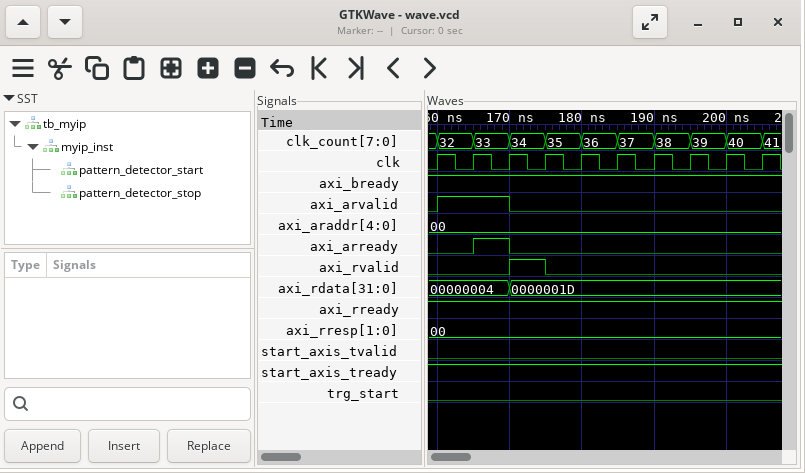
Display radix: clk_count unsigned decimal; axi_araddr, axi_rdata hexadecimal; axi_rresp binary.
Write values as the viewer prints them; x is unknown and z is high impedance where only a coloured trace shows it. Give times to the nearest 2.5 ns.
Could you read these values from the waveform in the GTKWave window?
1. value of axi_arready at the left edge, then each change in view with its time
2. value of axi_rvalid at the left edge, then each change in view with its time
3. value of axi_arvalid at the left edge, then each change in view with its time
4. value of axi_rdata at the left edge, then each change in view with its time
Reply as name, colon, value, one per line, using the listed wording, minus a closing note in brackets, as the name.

value of axi_arready at the left edge, then each change in view with its time: 0, 1 at 165 ns, 0 at 170 ns
value of axi_rvalid at the left edge, then each change in view with its time: 0, 1 at 170 ns, 0 at 175 ns
value of axi_arvalid at the left edge, then each change in view with its time: 0, 1 at 160 ns, 0 at 170 ns
value of axi_rdata at the left edge, then each change in view with its time: 00000004, 0000001D at 170 ns
